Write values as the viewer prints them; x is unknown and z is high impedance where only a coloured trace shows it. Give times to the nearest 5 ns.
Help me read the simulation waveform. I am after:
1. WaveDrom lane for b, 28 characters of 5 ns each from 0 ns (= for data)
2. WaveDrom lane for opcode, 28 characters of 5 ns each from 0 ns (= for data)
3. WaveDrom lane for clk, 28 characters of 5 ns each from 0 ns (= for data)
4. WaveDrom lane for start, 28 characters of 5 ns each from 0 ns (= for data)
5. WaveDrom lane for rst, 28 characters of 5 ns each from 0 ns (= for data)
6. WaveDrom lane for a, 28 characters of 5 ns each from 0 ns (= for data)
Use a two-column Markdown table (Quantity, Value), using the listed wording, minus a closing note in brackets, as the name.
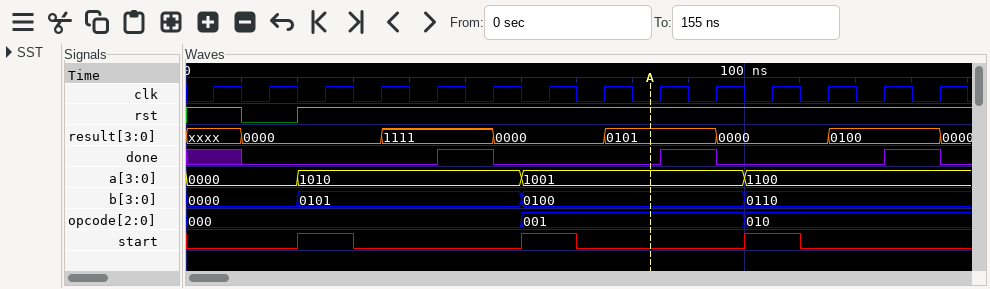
| Quantity | Value |
|---|---|
| WaveDrom lane for b, 28 characters of 5 ns each from 0 ns | {name: 'b', wave: '=...=.......=.......=.......', data: '0000 0101 0100 0110'} |
| WaveDrom lane for opcode, 28 characters of 5 ns each from 0 ns | {name: 'opcode', wave: '=...........=.......=.......', data: '000 001 010'} |
| WaveDrom lane for clk, 28 characters of 5 ns each from 0 ns | {name: 'clk', wave: '0101010101010101010101010101'} |
| WaveDrom lane for start, 28 characters of 5 ns each from 0 ns | {name: 'start', wave: '0...1.0.....1.0.....1.0.....'} |
| WaveDrom lane for rst, 28 characters of 5 ns each from 0 ns | {name: 'rst', wave: '1.0.1.......................'} |
| WaveDrom lane for a, 28 characters of 5 ns each from 0 ns | {name: 'a', wave: '=...=.......=.......=.......', data: '0000 1010 1001 1100'} |
